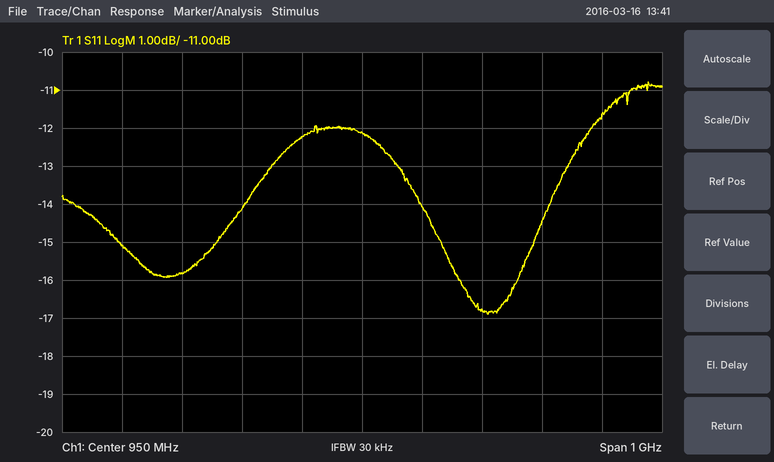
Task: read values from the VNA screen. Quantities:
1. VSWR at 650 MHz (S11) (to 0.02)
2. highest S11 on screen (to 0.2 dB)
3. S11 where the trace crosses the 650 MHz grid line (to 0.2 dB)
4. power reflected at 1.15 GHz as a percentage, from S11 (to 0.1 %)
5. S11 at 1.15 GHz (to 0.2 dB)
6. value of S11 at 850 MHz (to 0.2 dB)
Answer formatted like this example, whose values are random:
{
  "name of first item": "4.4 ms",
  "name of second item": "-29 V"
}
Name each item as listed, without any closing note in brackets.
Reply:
{
  "VSWR at 650 MHz (S11)": "1.38",
  "highest S11 on screen": "-10.8 dB",
  "S11 where the trace crosses the 650 MHz grid line": "-15.8 dB",
  "power reflected at 1.15 GHz as a percentage, from S11": "2.1 %",
  "S11 at 1.15 GHz": "-16.8 dB",
  "value of S11 at 850 MHz": "-12.2 dB"
}
